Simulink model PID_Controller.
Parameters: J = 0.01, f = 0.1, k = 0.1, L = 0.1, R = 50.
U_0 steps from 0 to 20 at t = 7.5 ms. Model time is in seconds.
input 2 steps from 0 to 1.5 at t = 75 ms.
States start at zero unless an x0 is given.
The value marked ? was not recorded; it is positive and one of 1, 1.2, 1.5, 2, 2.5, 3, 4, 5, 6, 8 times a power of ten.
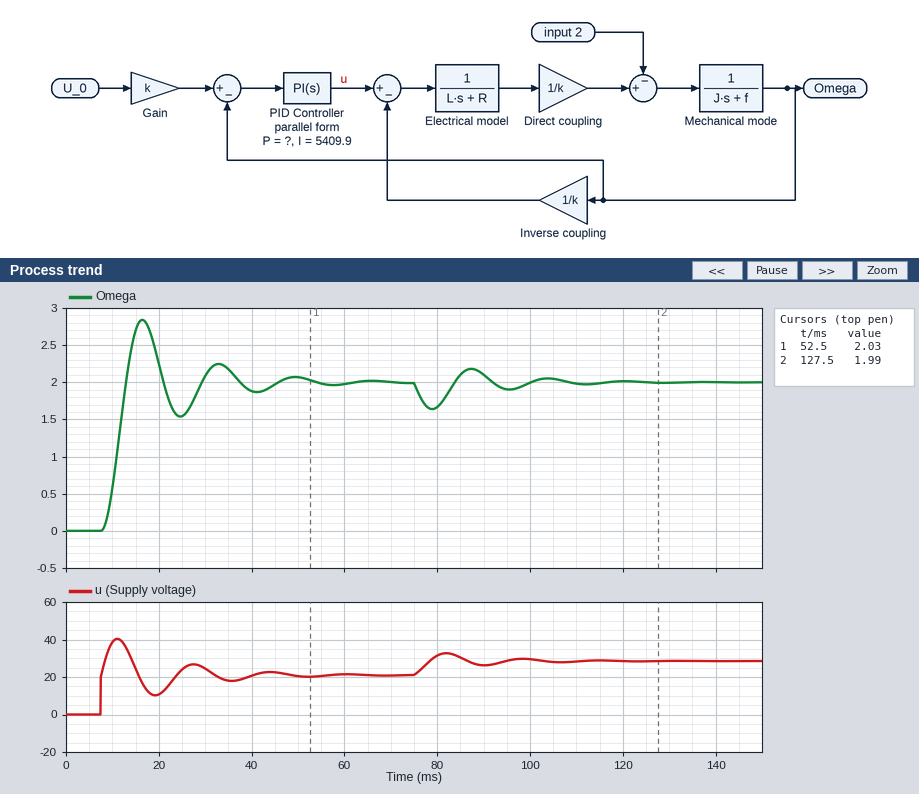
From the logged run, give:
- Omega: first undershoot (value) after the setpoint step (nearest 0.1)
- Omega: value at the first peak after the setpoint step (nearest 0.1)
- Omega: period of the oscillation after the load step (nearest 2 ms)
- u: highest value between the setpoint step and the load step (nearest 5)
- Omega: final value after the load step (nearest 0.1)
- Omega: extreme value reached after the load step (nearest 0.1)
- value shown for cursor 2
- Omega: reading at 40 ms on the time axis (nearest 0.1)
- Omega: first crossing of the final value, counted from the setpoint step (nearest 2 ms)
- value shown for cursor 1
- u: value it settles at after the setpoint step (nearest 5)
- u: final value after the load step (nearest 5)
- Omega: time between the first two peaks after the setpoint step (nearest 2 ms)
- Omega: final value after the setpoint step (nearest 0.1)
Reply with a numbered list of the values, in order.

1. 1.5
2. 2.8
3. 16 ms
4. 40
5. 2.0
6. 1.6
7. 1.99
8. 1.9
9. 6 ms
10. 2.03
11. 20
12. 30
13. 16 ms
14. 2.0
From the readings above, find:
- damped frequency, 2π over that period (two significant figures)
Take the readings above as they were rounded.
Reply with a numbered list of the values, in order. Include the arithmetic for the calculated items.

1. 2π / 16 = 0.39 rad/ms
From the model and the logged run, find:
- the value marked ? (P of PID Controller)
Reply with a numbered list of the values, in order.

1. 10
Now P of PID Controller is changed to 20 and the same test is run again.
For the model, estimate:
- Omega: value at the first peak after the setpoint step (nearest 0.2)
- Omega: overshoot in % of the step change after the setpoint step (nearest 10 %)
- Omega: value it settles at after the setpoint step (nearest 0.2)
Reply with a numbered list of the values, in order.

1. 2.6
2. 30 %
3. 2.0
